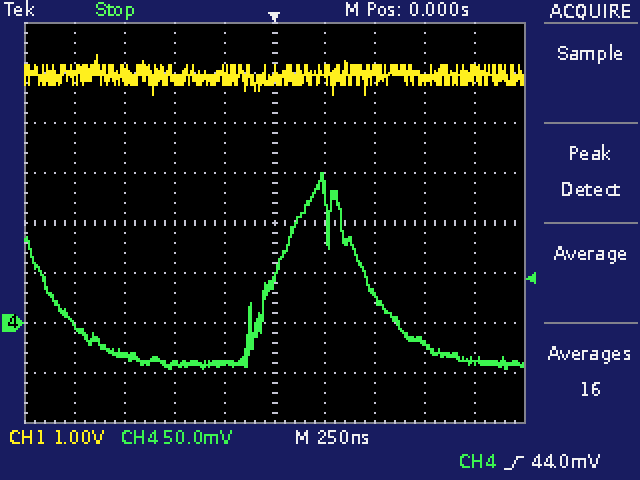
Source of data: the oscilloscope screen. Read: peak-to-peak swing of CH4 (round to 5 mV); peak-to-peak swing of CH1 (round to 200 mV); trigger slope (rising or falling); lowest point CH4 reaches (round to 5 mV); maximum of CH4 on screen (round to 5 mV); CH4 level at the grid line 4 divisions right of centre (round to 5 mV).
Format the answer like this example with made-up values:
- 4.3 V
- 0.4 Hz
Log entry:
- 195 mV
- 800 mV
- rising
- -45 mV
- 150 mV
- -40 mV
